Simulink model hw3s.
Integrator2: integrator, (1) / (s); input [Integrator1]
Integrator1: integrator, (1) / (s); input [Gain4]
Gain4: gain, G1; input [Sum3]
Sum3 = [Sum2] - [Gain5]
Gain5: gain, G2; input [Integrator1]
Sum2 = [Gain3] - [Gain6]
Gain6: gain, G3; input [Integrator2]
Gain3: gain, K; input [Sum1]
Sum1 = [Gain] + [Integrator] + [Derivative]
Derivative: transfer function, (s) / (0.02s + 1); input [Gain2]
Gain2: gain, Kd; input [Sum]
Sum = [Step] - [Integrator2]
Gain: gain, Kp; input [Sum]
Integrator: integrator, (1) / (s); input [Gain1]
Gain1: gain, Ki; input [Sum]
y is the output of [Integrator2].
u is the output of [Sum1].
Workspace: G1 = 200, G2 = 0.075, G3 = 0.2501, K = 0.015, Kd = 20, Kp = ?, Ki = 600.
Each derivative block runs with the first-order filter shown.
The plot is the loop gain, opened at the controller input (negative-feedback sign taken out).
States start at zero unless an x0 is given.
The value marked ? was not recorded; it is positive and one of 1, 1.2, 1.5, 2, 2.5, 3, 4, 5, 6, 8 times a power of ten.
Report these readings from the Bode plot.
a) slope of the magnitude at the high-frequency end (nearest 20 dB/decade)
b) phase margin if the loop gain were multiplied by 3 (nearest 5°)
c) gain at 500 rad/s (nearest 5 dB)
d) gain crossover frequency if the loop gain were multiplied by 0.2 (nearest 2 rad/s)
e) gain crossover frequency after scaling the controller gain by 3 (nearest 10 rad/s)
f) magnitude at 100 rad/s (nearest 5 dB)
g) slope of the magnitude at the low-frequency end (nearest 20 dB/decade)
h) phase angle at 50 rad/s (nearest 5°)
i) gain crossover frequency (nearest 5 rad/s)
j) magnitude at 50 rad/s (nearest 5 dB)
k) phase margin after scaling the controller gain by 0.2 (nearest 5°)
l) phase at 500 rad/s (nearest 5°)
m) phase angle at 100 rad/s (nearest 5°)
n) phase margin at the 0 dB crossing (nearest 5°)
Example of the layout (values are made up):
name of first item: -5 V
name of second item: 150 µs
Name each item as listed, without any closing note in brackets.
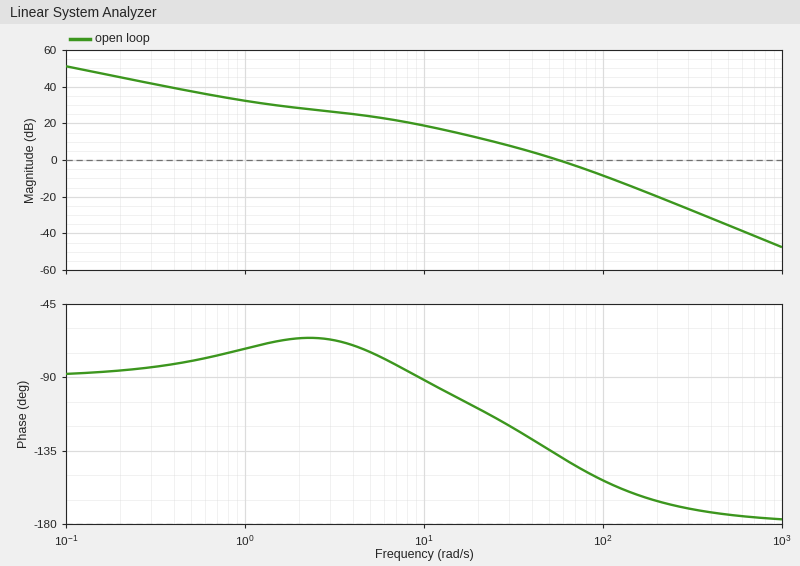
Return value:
slope of the magnitude at the high-frequency end: -40 dB/decade
phase margin if the loop gain were multiplied by 3: 25°
gain at 500 rad/s: -35 dB
gain crossover frequency if the loop gain were multiplied by 0.2: 16 rad/s
gain crossover frequency after scaling the controller gain by 3: 110 rad/s
magnitude at 100 rad/s: -10 dB
slope of the magnitude at the low-frequency end: -20 dB/decade
phase angle at 50 rad/s: -135°
gain crossover frequency: 55 rad/s
magnitude at 50 rad/s: 0 dB
phase margin after scaling the controller gain by 0.2: 75°
phase at 500 rad/s: -175°
phase angle at 100 rad/s: -155°
phase margin at the 0 dB crossing: 40°
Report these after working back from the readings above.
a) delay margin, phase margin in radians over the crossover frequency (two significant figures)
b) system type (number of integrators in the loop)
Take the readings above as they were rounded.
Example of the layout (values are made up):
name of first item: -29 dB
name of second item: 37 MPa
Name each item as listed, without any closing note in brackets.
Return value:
delay margin, phase margin in radians over the crossover frequency: 0.013 s
system type: 1
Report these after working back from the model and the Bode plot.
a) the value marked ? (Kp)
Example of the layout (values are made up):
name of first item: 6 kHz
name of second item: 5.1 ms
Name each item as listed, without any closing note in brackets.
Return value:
the value marked ?: 400
